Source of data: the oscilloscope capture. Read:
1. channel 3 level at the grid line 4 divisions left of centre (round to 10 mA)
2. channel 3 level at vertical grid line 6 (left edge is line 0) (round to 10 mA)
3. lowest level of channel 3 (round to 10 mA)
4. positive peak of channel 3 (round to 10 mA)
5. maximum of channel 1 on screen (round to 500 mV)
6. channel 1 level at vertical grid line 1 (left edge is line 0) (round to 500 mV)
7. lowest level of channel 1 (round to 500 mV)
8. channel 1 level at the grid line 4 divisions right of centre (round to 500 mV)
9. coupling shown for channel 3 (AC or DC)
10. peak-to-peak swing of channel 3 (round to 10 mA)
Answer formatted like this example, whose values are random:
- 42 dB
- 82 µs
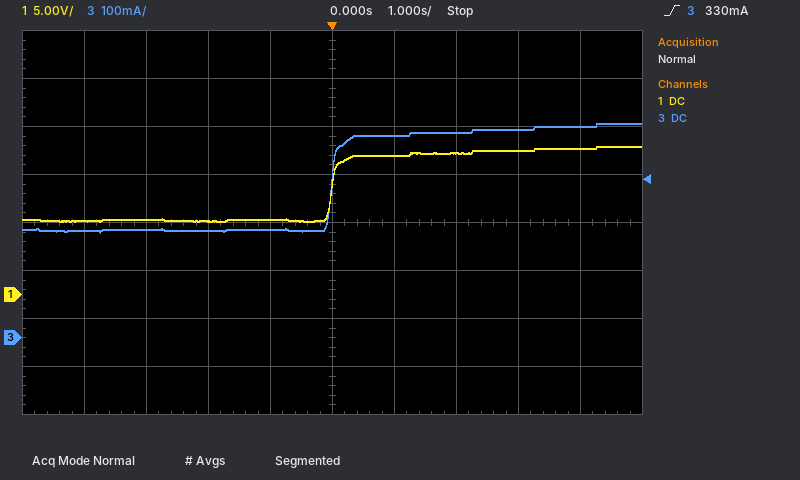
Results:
- 220 mA
- 420 mA
- 220 mA
- 450 mA
- 15.5 V
- 7.5 V
- 7.5 V
- 15.0 V
- DC
- 230 mA
